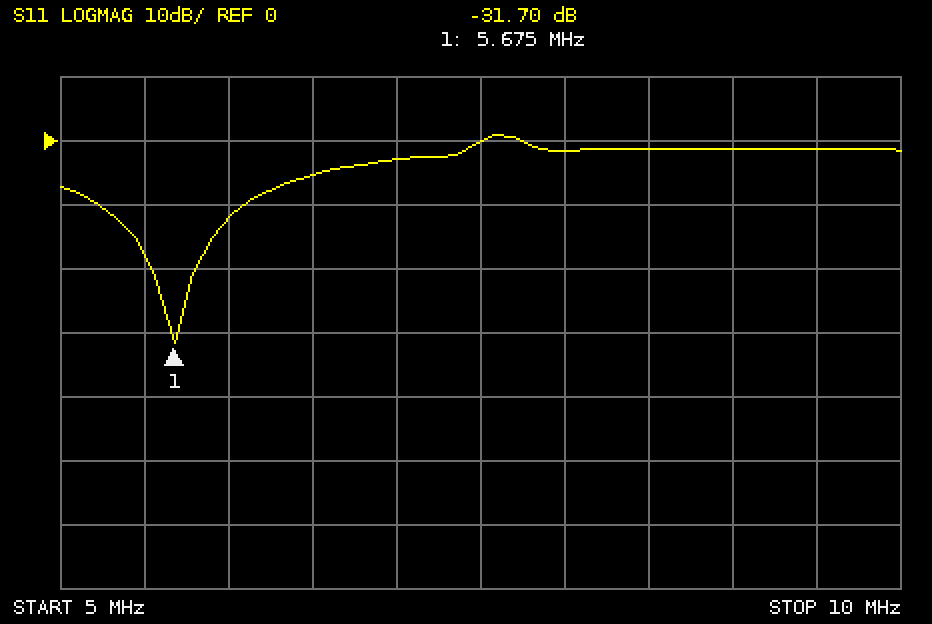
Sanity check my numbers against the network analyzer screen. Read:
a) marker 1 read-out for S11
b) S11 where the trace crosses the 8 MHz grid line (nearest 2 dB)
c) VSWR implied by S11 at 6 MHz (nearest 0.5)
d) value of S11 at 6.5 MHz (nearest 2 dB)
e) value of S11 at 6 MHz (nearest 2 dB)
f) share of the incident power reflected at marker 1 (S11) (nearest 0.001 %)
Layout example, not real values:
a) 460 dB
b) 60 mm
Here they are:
a) -31.70 dB
b) -2 dB
c) 1.5
d) -6 dB
e) -12 dB
f) 0.068 %
